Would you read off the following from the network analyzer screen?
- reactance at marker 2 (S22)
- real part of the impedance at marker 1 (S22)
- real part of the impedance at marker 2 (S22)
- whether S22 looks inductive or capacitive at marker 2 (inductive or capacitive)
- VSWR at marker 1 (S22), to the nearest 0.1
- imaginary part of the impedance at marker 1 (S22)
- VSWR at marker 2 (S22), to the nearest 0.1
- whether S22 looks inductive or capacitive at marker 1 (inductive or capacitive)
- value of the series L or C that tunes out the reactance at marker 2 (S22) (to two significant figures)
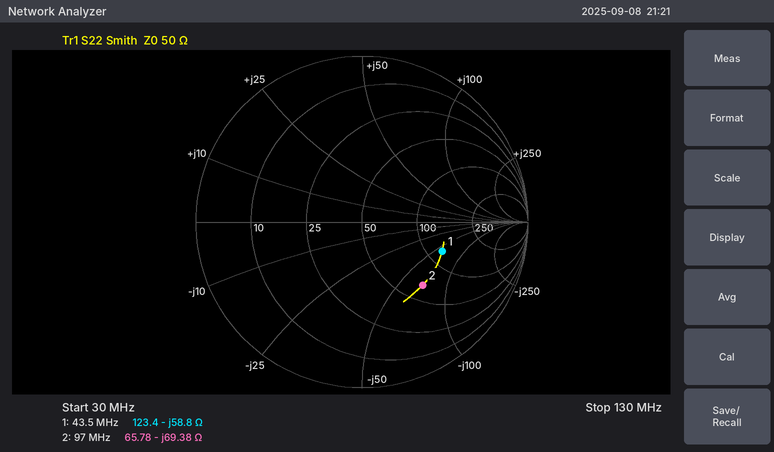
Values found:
-69.38 Ω
123.4 Ω
65.78 Ω
capacitive
3.1
-58.8 Ω
3.2
capacitive
110 nH
